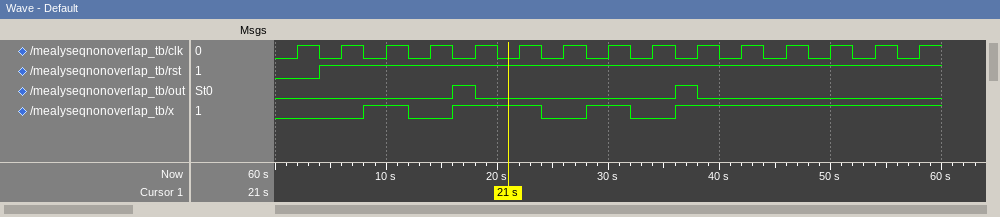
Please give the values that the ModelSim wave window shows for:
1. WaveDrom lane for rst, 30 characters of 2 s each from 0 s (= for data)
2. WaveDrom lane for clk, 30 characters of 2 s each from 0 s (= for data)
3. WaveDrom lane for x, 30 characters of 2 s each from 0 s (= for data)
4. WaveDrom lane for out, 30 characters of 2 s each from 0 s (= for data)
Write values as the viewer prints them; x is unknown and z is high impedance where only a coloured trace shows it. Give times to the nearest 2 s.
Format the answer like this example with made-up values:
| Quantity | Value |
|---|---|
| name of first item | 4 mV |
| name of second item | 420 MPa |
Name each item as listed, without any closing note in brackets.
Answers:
| Quantity | Value |
|---|---|
| WaveDrom lane for rst, 30 characters of 2 s each from 0 s | {name: 'rst', wave: '0.1...........................'} |
| WaveDrom lane for clk, 30 characters of 2 s each from 0 s | {name: 'clk', wave: '010101010101010101010101010101'} |
| WaveDrom lane for x, 30 characters of 2 s each from 0 s | {name: 'x', wave: '0...1.0.1...0.1.0.1...........'} |
| WaveDrom lane for out, 30 characters of 2 s each from 0 s | {name: 'out', wave: '0.......10........10..........'} |
